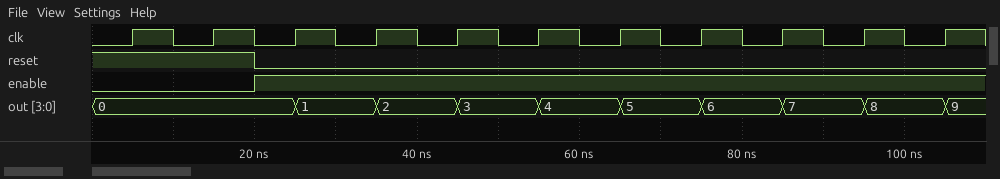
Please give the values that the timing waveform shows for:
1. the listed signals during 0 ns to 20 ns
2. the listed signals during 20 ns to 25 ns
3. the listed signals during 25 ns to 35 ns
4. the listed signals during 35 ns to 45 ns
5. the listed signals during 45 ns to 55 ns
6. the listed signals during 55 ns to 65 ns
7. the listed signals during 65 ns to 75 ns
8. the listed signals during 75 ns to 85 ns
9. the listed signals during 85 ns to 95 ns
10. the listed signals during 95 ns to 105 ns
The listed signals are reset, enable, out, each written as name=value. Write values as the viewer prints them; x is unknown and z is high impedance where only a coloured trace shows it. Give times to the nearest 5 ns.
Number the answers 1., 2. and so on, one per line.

1. reset=1, enable=0, out=0
2. reset=0, enable=1, out=0
3. reset=0, enable=1, out=1
4. reset=0, enable=1, out=2
5. reset=0, enable=1, out=3
6. reset=0, enable=1, out=4
7. reset=0, enable=1, out=5
8. reset=0, enable=1, out=6
9. reset=0, enable=1, out=7
10. reset=0, enable=1, out=8
